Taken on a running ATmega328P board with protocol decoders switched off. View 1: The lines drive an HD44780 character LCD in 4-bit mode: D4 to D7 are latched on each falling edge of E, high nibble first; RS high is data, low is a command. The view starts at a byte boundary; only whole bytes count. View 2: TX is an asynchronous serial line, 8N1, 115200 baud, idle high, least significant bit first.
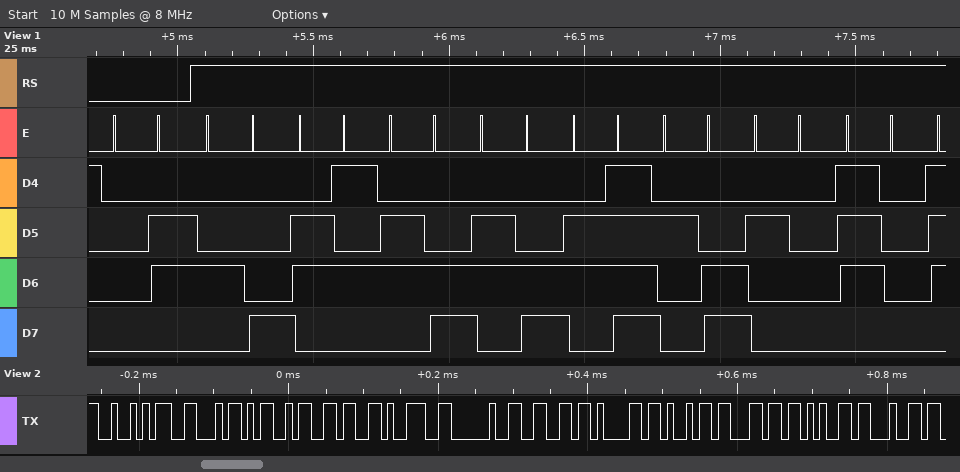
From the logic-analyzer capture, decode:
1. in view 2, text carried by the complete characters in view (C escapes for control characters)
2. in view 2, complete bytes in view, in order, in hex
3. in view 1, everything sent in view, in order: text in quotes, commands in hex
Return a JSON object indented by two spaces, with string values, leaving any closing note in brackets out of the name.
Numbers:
{
  "in view 2, text carried by the complete characters in view": "\"RFM69 failed\"",
  "in view 2, complete bytes in view, in order, in hex": "52 46 4D 36 39 20 66 61 69 6C 65 64",
  "in view 1, everything sent in view, in order: text in quotes, commands in hex": "0x06 \"Hello, p\""
}
